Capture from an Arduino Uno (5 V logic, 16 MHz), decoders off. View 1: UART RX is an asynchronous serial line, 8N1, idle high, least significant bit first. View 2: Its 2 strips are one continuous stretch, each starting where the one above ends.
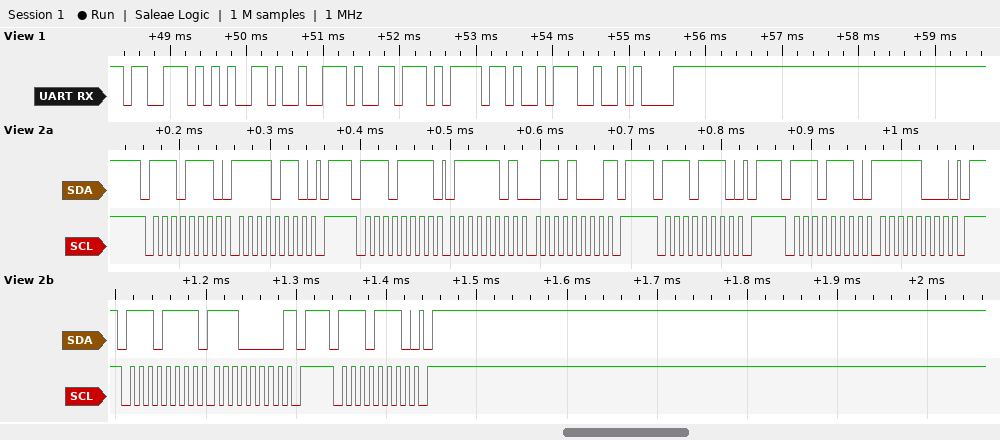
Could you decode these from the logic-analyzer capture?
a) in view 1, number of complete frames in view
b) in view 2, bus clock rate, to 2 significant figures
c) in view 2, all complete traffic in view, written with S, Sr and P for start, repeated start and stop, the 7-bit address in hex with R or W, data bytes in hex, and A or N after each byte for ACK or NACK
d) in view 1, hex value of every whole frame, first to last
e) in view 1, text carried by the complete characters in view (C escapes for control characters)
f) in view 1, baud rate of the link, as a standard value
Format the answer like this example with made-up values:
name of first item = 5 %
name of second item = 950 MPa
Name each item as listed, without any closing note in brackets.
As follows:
in view 1, number of complete frames in view = 7
in view 2, bus clock rate, to 2 significant figures = 100 kHz
in view 2, all complete traffic in view, written with S, Sr and P for start, repeated start and stop, the 7-bit address in hex with R or W, data bytes in hex, and A or N after each byte for ACK or NACK = S 77W A F6 A P S 77R A 7D A 68 N P S 77W A P S 77W A F8 A P S 77R A E0 N P S 77W A P
in view 1, hex value of every whole frame, first to last = 0x73 0x65 0x72 0x76 0x6F 0x3A 0x0A
in view 1, text carried by the complete characters in view = "servo:\n"
in view 1, baud rate of the link, as a standard value = 9600 baud
